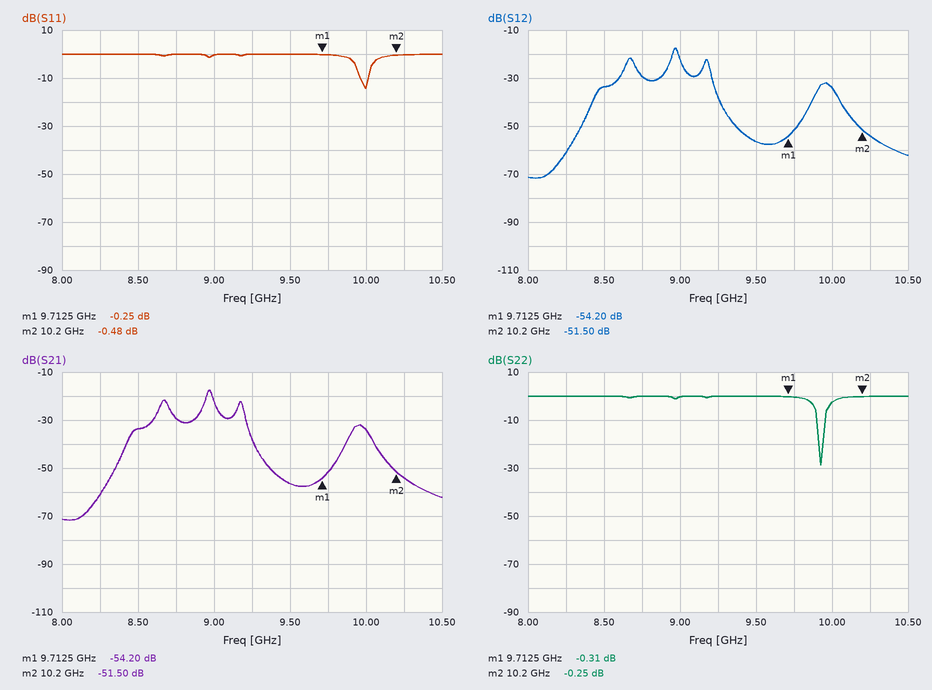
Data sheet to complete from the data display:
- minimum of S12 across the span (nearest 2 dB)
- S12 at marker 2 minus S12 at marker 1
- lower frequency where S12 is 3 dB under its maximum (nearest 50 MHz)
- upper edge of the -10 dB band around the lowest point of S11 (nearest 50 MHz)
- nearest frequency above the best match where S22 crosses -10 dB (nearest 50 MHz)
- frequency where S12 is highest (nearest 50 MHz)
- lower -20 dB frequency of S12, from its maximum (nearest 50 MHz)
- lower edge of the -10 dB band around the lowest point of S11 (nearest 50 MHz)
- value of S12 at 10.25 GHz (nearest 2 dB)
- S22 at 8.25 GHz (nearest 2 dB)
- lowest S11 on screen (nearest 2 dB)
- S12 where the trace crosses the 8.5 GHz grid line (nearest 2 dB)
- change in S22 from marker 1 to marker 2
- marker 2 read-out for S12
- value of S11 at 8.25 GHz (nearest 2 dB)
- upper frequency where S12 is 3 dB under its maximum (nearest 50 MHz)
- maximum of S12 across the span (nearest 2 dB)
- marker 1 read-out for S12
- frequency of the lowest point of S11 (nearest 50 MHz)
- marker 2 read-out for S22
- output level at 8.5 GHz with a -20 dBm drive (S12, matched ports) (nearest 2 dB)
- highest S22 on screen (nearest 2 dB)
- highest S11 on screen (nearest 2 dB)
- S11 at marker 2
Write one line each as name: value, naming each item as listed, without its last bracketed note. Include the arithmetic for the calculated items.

minimum of S12 across the span: -72 dB
S12 at marker 2 minus S12 at marker 1: -51.5 − (-54.2) = 2.70 dB
lower frequency where S12 is 3 dB under its maximum: 8.95 GHz
upper edge of the -10 dB band around the lowest point of S11: 10.00 GHz
nearest frequency above the best match where S22 crosses -10 dB: 9.95 GHz
frequency where S12 is highest: 8.95 GHz
lower -20 dB frequency of S12, from its maximum: 8.45 GHz
lower edge of the -10 dB band around the lowest point of S11: 9.95 GHz
value of S12 at 10.25 GHz: -54 dB
S22 at 8.25 GHz: 0 dB
lowest S11 on screen: -14 dB
S12 where the trace crosses the 8.5 GHz grid line: -34 dB
change in S22 from marker 1 to marker 2: -0.25 − (-0.31) = 0.06 dB
marker 2 read-out for S12: -51.50 dB
value of S11 at 8.25 GHz: 0 dB
upper frequency where S12 is 3 dB under its maximum: 9.00 GHz
maximum of S12 across the span: -18 dB
marker 1 read-out for S12: -54.20 dB
frequency of the lowest point of S11: 10.00 GHz
marker 2 read-out for S22: -0.25 dB
output level at 8.5 GHz with a -20 dBm drive (S12, matched ports): -20 dBm + (-34 dB) = -54 dBm
highest S22 on screen: 0 dB
highest S11 on screen: 0 dB
S11 at marker 2: -0.48 dB
